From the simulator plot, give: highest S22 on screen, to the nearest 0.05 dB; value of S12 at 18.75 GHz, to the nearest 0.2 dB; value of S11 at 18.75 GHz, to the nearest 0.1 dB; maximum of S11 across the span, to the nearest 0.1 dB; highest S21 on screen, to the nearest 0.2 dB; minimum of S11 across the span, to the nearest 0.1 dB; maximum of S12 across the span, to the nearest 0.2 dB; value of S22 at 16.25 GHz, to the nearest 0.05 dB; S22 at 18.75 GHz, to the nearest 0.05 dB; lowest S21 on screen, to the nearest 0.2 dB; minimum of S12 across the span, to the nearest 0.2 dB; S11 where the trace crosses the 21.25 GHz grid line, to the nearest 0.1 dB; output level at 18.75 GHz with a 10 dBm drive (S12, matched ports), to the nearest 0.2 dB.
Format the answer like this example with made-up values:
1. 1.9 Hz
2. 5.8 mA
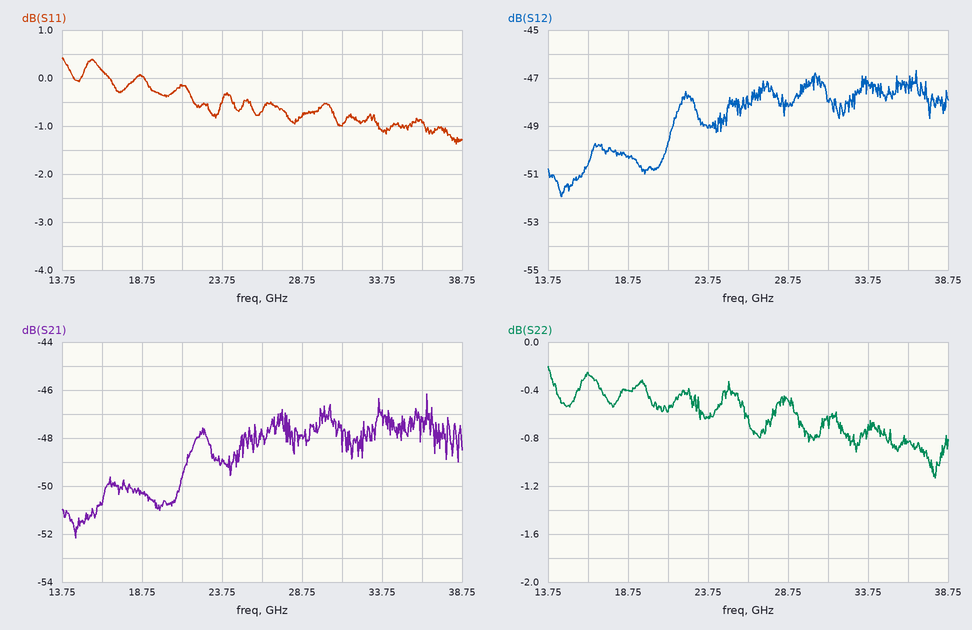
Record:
1. -0.20 dB
2. -50.2 dB
3. 0.0 dB
4. 0.4 dB
5. -46.2 dB
6. -1.4 dB
7. -46.6 dB
8. -0.25 dB
9. -0.40 dB
10. -52.2 dB
11. -52.0 dB
12. -0.2 dB
13. -40.2 dBm
